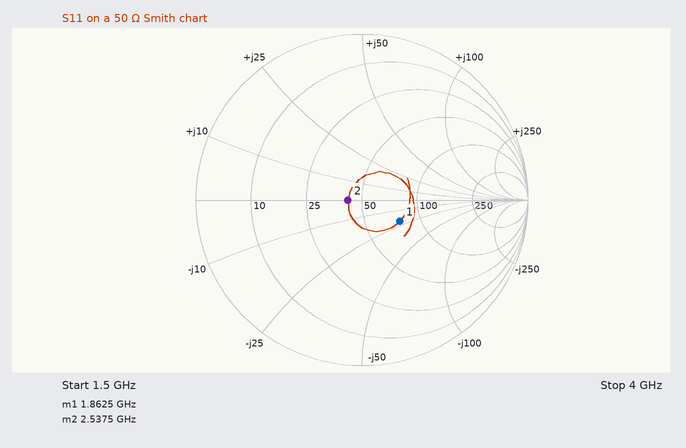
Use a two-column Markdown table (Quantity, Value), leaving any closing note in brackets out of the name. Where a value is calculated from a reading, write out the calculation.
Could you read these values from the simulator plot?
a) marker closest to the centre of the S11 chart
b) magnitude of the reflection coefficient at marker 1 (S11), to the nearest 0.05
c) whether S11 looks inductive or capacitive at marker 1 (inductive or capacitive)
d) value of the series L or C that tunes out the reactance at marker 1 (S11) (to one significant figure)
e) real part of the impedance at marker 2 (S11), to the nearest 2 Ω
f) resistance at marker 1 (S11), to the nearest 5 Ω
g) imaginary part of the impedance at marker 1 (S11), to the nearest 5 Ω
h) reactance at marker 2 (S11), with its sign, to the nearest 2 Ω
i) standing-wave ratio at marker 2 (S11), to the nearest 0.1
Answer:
| Quantity | Value |
|---|---|
| marker closest to the centre of the S11 chart | marker 2 |
| magnitude of the reflection coefficient at marker 1 (S11), to the nearest 0.05 | 0.25 |
| whether S11 looks inductive or capacitive at marker 1 | capacitive |
| value of the series L or C that tunes out the reactance at marker 1 (S11) | L = 20 Ω/(2π × 1.8625 GHz) ≈ 2 nH |
| real part of the impedance at marker 2 (S11), to the nearest 2 Ω | 42 Ω |
| resistance at marker 1 (S11), to the nearest 5 Ω | 75 Ω |
| imaginary part of the impedance at marker 1 (S11), to the nearest 5 Ω | -20 Ω |
| reactance at marker 2 (S11), with its sign, to the nearest 2 Ω | 0 Ω |
| standing-wave ratio at marker 2 (S11), to the nearest 0.1 | 1.2 |
